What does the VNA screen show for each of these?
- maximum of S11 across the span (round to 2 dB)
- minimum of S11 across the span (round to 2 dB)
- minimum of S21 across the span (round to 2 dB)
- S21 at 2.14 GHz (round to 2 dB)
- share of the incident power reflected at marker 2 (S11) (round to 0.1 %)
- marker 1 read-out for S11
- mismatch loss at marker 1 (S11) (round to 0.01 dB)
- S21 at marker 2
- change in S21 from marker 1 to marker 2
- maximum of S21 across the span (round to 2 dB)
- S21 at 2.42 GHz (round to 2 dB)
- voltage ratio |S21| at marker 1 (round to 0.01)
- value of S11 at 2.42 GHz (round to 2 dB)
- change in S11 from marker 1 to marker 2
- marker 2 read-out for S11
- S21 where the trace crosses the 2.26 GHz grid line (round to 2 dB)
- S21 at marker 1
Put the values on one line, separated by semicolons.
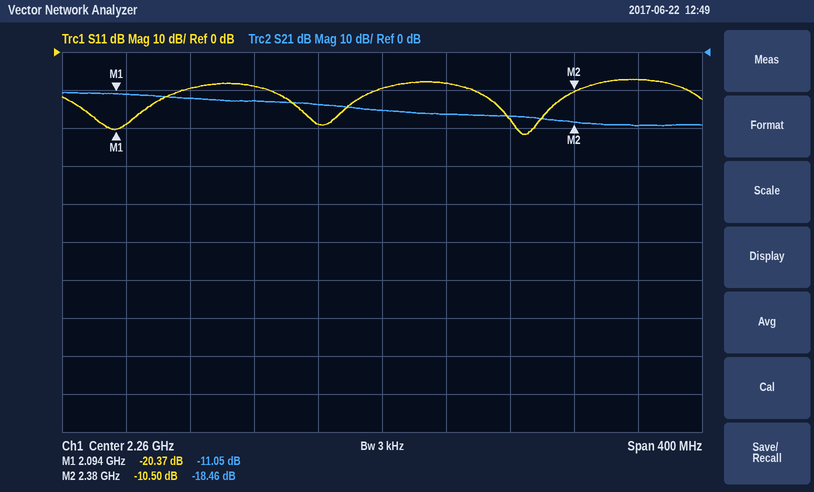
-8 dB; -22 dB; -20 dB; -12 dB; 8.9 %; -20.37 dB; 0.04 dB; -18.46 dB; -7.41 dB; -10 dB; -20 dB; 0.28; -8 dB; 9.87 dB; -10.50 dB; -16 dB; -11.05 dB
